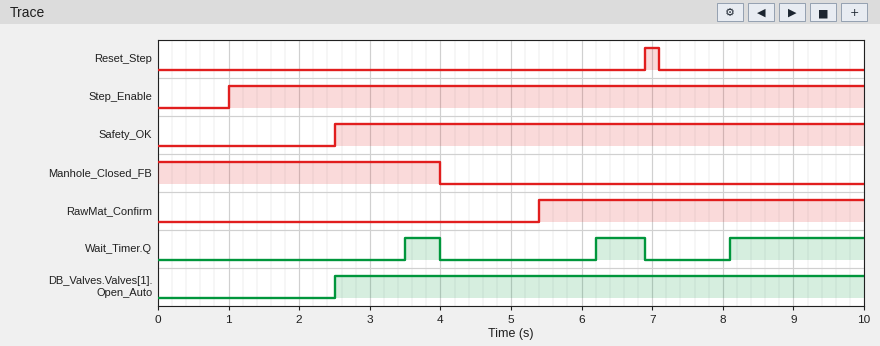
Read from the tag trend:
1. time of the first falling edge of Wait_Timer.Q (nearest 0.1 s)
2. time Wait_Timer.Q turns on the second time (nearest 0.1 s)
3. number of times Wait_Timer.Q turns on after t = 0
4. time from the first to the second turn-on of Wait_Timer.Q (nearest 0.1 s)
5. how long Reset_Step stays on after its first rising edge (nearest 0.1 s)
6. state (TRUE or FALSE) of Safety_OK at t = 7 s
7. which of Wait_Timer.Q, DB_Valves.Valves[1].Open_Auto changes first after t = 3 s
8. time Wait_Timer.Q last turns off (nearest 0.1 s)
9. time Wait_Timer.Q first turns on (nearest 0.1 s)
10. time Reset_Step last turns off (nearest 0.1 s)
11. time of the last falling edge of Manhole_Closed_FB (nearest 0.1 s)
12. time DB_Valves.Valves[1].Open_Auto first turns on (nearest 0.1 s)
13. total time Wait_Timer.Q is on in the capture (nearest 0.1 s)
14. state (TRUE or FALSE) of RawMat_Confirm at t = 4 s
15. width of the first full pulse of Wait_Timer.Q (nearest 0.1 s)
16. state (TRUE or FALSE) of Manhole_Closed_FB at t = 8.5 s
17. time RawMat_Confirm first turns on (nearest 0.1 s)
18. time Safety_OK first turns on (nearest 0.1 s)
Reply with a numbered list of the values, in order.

1. 4.0 s
2. 6.2 s
3. 3
4. 2.7 s
5. 0.2 s
6. TRUE
7. Wait_Timer.Q
8. 6.9 s
9. 3.5 s
10. 7.1 s
11. 4.0 s
12. 2.5 s
13. 3.1 s
14. FALSE
15. 0.5 s
16. FALSE
17. 5.4 s
18. 2.5 s
